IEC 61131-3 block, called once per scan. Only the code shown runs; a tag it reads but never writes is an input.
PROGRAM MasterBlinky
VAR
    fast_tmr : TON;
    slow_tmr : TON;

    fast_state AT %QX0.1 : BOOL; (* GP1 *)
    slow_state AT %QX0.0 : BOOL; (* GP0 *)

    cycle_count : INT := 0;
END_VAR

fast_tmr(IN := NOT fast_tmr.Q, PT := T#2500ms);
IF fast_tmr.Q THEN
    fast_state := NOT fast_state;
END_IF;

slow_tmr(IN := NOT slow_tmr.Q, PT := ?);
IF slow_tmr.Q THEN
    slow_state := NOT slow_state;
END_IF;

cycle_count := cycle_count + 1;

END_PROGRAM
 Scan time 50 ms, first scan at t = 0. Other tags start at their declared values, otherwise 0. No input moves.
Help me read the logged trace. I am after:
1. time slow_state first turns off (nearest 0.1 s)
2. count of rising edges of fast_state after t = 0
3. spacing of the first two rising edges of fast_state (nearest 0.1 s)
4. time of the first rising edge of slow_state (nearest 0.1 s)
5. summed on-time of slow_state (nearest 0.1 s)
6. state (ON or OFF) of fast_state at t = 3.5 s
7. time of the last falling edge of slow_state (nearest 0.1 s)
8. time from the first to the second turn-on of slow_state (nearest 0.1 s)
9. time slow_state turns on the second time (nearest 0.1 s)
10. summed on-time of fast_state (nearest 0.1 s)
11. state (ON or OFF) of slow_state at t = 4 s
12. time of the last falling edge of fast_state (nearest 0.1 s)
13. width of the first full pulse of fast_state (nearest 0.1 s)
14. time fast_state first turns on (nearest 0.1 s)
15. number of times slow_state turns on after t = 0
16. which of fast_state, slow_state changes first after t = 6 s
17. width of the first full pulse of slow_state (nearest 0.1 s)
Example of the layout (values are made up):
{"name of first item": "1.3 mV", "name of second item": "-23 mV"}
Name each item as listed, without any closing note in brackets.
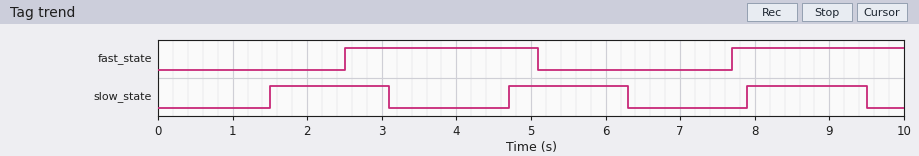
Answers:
{"time slow_state first turns off": "3.1 s", "count of rising edges of fast_state after t = 0": "2", "spacing of the first two rising edges of fast_state": "5.2 s", "time of the first rising edge of slow_state": "1.5 s", "summed on-time of slow_state": "4.8 s", "state (ON or OFF) of fast_state at t = 3.5 s": "ON", "time of the last falling edge of slow_state": "9.5 s", "time from the first to the second turn-on of slow_state": "3.2 s", "time slow_state turns on the second time": "4.7 s", "summed on-time of fast_state": "4.9 s", "state (ON or OFF) of slow_state at t = 4 s": "OFF", "time of the last falling edge of fast_state": "5.1 s", "width of the first full pulse of fast_state": "2.6 s", "time fast_state first turns on": "2.5 s", "number of times slow_state turns on after t = 0": "3", "which of fast_state, slow_state changes first after t = 6 s": "slow_state", "width of the first full pulse of slow_state": "1.6 s"}
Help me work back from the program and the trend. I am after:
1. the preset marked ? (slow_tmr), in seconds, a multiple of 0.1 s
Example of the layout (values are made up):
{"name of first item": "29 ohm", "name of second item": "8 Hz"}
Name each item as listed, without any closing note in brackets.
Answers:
{"the preset marked ? (slow_tmr), in seconds, a multiple of 0.1 s": "1.5 s"}
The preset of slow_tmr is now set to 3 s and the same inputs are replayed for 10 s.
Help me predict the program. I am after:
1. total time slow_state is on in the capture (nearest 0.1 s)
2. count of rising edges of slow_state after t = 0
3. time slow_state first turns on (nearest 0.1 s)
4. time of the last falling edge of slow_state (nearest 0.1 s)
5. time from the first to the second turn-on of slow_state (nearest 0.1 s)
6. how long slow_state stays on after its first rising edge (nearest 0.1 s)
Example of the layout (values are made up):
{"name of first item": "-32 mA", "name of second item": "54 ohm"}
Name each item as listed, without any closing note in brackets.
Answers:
{"total time slow_state is on in the capture": "3.9 s", "count of rising edges of slow_state after t = 0": "2", "time slow_state first turns on": "3.0 s", "time of the last falling edge of slow_state": "6.1 s", "time from the first to the second turn-on of slow_state": "6.2 s", "how long slow_state stays on after its first rising edge": "3.1 s"}
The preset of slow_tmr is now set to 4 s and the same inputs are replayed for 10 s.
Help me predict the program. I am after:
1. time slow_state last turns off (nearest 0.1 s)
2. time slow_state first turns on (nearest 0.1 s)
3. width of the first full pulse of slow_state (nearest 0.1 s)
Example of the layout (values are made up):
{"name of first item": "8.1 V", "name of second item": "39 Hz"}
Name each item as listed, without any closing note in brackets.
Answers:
{"time slow_state last turns off": "8.1 s", "time slow_state first turns on": "4.0 s", "width of the first full pulse of slow_state": "4.1 s"}
